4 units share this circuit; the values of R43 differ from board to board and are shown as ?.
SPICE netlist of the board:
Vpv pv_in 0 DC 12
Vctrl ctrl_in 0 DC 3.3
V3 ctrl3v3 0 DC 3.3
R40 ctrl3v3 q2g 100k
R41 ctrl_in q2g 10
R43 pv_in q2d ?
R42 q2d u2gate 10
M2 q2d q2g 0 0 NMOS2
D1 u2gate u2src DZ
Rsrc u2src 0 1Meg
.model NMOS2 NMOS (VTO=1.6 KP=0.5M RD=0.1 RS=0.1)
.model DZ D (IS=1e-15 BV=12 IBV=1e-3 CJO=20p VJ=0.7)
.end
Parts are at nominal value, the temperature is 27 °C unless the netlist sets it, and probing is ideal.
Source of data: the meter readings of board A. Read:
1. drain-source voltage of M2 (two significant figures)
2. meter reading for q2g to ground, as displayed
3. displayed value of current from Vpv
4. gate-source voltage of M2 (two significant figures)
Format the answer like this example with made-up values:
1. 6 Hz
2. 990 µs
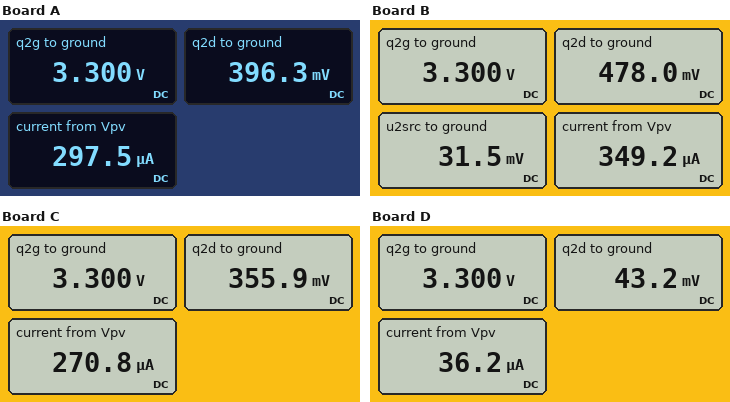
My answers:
1. 400 mV
2. 3.300 V
3. 297.5 µA
4. 3.3 V
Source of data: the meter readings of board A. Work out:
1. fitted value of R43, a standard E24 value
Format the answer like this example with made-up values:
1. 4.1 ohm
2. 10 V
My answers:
1. 39 kΩ
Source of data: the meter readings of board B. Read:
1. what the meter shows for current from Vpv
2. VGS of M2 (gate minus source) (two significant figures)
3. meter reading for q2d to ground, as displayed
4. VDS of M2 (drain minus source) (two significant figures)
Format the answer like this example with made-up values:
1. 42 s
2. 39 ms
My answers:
1. 349.2 µA
2. 3.3 V
3. 478.0 mV
4. 480 mV
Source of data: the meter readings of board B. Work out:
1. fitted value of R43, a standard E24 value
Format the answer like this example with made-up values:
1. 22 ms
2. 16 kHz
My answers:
1. 33 kΩ
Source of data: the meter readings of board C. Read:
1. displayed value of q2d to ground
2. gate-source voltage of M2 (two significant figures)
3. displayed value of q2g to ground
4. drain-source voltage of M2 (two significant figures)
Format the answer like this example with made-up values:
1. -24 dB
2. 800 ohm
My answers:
1. 355.9 mV
2. 3.3 V
3. 3.300 V
4. 360 mV
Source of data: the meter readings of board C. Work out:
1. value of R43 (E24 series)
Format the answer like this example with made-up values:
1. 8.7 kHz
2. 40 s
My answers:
1. 43 kΩ
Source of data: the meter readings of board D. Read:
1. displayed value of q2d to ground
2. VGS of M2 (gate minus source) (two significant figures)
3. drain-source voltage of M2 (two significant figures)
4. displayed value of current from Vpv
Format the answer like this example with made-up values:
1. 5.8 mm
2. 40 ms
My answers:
1. 43.2 mV
2. 3.3 V
3. 43 mV
4. 36.2 µA
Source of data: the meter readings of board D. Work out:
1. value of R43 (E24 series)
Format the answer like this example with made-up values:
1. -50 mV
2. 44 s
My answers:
1. 330 kΩ
